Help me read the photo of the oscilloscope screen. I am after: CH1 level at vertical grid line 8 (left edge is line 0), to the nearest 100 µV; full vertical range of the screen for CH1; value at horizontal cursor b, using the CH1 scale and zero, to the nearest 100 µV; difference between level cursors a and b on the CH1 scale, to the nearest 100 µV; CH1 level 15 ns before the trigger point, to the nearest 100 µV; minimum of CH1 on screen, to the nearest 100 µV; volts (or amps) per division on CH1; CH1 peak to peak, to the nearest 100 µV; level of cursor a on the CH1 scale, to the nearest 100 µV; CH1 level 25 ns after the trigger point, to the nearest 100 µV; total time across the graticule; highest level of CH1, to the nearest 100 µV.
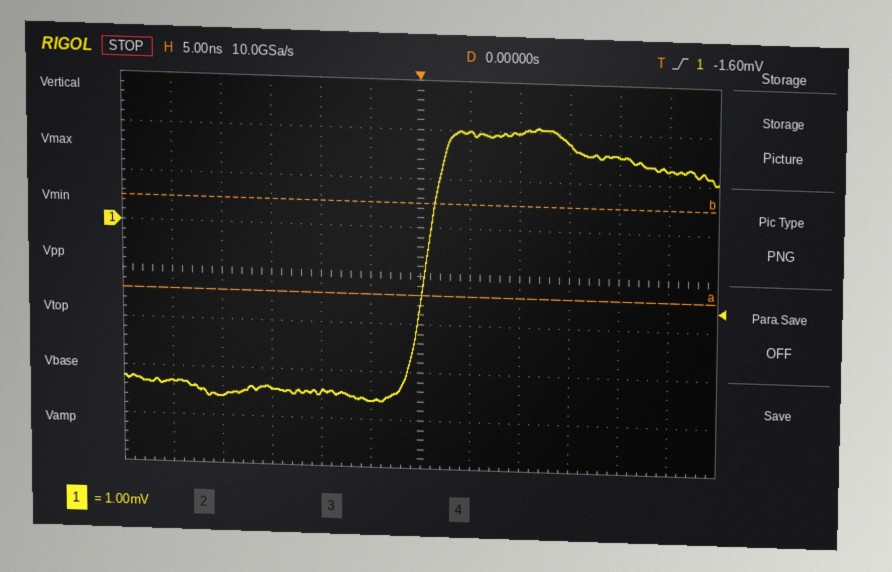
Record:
2.0 mV
8 mV
500 µV
1.9 mV
-3.4 mV
-3.6 mV
1 mV
5.7 mV
-1.4 mV
1.3 mV
60 ns
2.1 mV
